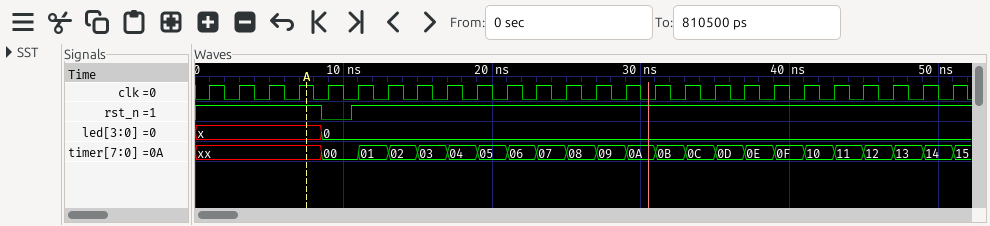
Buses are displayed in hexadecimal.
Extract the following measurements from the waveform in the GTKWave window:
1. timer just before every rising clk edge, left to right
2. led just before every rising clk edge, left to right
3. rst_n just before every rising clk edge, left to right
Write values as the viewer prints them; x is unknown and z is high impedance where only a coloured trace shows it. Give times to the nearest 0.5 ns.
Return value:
xx, xx, xx, xx, 00, 00, 01, 02, 03, 04, 05, 06, 07, 08, 09, 0A, 0B, 0C, 0D, 0E, 0F, 10, 11, 12, 13, 14
x, x, x, x, 0, 0, 0, 0, 0, 0, 0, 0, 0, 0, 0, 0, 0, 0, 0, 0, 0, 0, 0, 0, 0, 0
1 1 1 1 0 1 1 1 1 1 1 1 1 1 1 1 1 1 1 1 1 1 1 1 1 1
